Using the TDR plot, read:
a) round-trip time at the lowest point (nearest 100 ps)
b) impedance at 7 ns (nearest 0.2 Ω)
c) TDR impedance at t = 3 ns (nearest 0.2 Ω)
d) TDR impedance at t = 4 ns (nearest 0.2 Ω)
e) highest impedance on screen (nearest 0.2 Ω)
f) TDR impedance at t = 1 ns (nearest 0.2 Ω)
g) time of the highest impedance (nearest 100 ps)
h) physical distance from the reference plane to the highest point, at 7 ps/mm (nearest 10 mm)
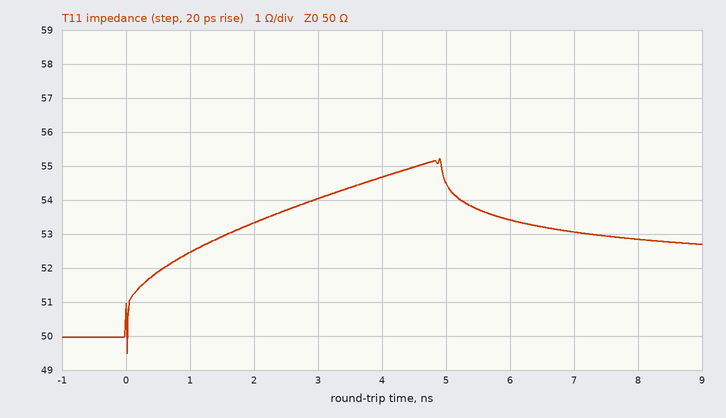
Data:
0.0 ns
53.0 Ω
54.0 Ω
54.6 Ω
55.2 Ω
52.4 Ω
4.9 ns
350 mm
